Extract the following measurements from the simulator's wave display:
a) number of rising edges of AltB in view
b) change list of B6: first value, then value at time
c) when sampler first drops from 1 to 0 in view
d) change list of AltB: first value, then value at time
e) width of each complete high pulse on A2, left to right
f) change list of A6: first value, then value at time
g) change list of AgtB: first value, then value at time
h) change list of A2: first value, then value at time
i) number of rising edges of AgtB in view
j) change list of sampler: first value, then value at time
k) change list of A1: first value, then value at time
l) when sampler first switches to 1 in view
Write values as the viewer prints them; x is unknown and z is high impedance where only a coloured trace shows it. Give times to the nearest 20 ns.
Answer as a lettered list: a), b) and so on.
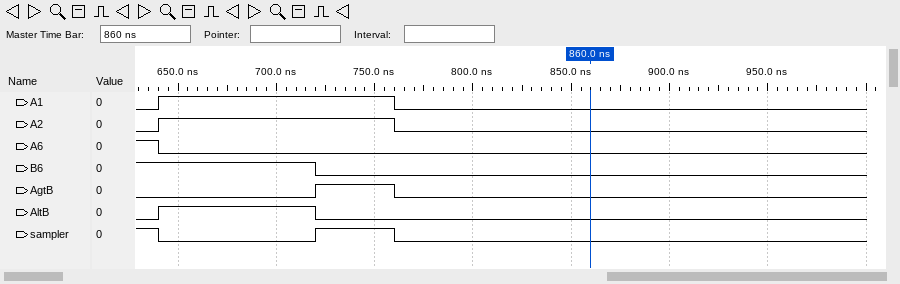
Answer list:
a) 1
b) 1, 0 at 720 ns
c) 640 ns
d) 0, 1 at 640 ns, 0 at 720 ns
e) 120 ns
f) 1, 0 at 640 ns
g) 0, 1 at 720 ns, 0 at 760 ns
h) 0, 1 at 640 ns, 0 at 760 ns
i) 1
j) 1, 0 at 640 ns, 1 at 720 ns, 0 at 760 ns
k) 0, 1 at 640 ns, 0 at 760 ns
l) 720 ns
